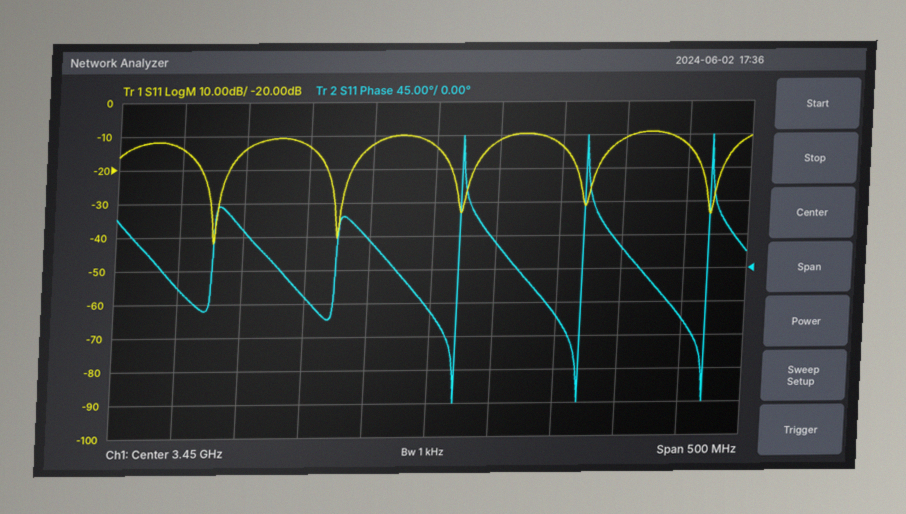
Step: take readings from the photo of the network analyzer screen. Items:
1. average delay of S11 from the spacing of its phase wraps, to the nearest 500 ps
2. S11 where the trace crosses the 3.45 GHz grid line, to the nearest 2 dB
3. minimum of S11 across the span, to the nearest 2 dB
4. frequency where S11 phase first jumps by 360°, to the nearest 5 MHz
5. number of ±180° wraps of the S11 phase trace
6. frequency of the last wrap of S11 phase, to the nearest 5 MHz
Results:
10.0 ns
-14 dB
-42 dB
3.470 GHz
3
3.670 GHz
